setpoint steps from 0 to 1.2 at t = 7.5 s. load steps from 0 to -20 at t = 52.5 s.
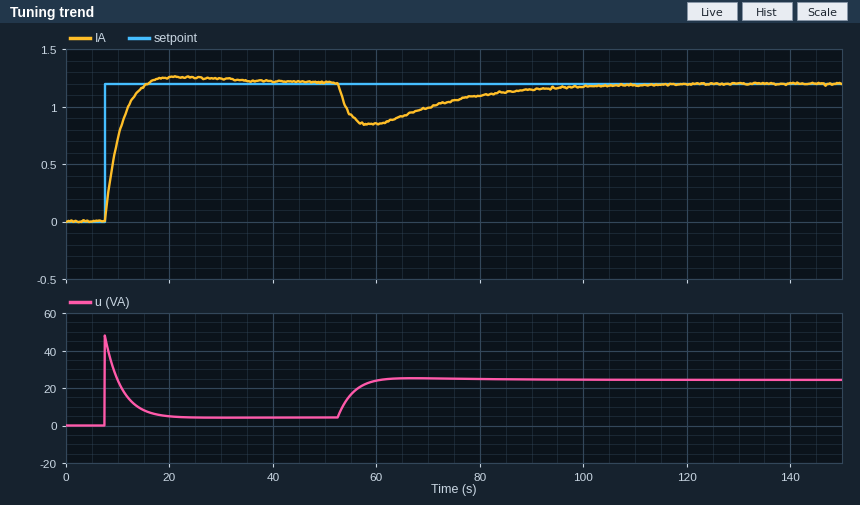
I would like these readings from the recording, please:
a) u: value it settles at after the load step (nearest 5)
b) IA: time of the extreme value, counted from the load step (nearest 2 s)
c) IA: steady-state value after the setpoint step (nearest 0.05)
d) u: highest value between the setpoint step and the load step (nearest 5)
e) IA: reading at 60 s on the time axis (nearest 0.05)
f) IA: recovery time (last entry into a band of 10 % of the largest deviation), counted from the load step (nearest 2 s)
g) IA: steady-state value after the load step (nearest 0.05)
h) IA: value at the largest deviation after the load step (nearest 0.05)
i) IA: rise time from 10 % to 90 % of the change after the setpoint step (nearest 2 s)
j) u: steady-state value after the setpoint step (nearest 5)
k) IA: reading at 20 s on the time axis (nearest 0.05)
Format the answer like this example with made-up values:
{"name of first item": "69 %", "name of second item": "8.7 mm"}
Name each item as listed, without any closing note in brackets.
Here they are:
{"u: value it settles at after the load step": "25", "IA: time of the extreme value, counted from the load step": "6 s", "IA: steady-state value after the setpoint step": "1.20", "u: highest value between the setpoint step and the load step": "50", "IA: reading at 60 s on the time axis": "0.85", "IA: recovery time (last entry into a band of 10 % of the largest deviation), counted from the load step": "42 s", "IA: steady-state value after the load step": "1.20", "IA: value at the largest deviation after the load step": "0.85", "IA: rise time from 10 % to 90 % of the change after the setpoint step": "6 s", "u: steady-state value after the setpoint step": "5", "IA: reading at 20 s on the time axis": "1.25"}
